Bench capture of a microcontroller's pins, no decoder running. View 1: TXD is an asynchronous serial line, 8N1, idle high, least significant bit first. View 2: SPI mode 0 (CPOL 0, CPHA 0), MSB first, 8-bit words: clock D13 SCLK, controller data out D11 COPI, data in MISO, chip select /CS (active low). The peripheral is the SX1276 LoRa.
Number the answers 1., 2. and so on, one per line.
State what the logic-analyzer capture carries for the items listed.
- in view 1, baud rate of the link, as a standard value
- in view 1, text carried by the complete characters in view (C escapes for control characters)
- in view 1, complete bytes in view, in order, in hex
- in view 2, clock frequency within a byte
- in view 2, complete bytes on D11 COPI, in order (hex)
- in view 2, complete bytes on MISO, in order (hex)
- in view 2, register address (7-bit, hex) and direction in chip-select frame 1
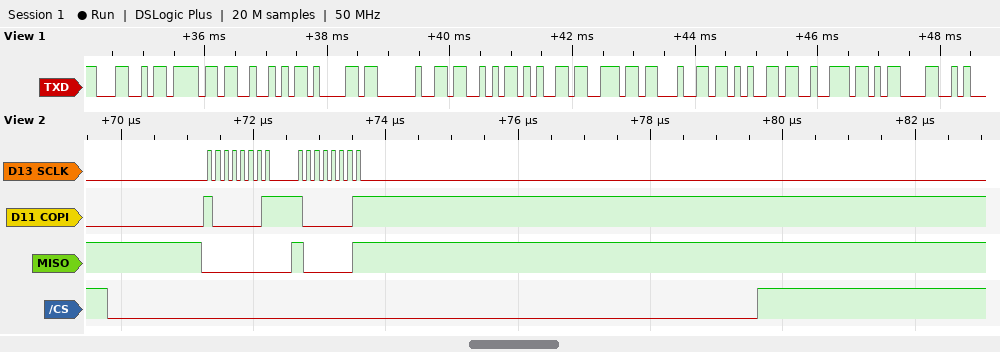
1. 9600 baud
2. "LoRa Sender\r"
3. 0x4C 0x6F 0x52 0x61 0x20 0x53 0x65 0x6E 0x64 0x65 0x72 0x0D
4. 8 MHz
5. 0x81 0x81
6. 0x00 0x81
7. 0x01 write
